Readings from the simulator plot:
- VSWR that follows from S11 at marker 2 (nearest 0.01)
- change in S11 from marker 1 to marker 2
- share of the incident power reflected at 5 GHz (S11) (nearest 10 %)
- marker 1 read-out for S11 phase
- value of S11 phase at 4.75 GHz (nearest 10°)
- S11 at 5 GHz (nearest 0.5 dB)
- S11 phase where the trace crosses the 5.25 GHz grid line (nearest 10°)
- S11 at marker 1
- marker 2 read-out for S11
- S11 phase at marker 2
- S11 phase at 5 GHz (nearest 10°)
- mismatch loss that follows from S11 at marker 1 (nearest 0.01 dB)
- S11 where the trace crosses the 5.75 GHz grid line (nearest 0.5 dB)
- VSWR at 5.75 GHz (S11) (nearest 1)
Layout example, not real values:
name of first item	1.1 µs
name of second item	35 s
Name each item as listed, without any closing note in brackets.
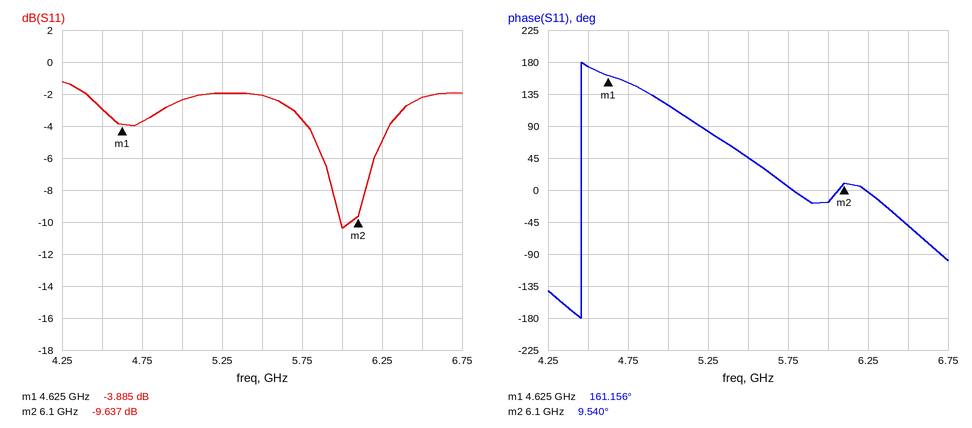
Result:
VSWR that follows from S11 at marker 2	1.98
change in S11 from marker 1 to marker 2	-5.752 dB
share of the incident power reflected at 5 GHz (S11)	60 %
marker 1 read-out for S11 phase	161.156°
value of S11 phase at 4.75 GHz	150°
S11 at 5 GHz	-2.5 dB
S11 phase where the trace crosses the 5.25 GHz grid line	80°
S11 at marker 1	-3.885 dB
marker 2 read-out for S11	-9.637 dB
S11 phase at marker 2	9.540°
S11 phase at 5 GHz	120°
mismatch loss that follows from S11 at marker 1	2.28 dB
S11 where the trace crosses the 5.75 GHz grid line	-3.5 dB
VSWR at 5.75 GHz (S11)	5
